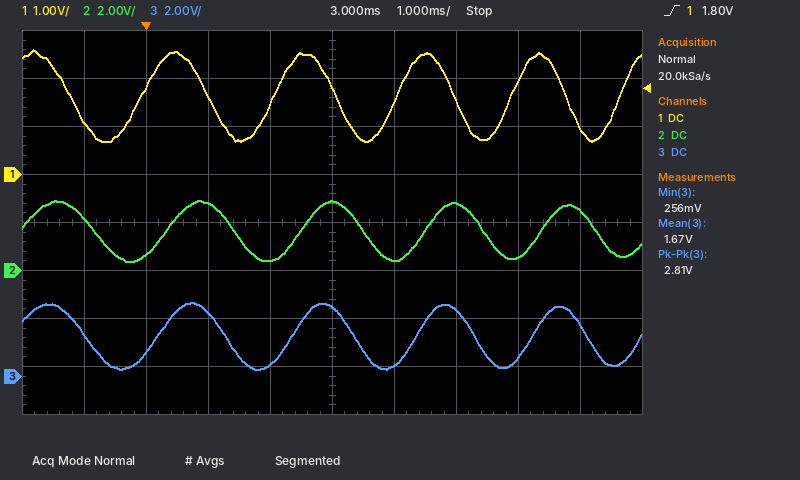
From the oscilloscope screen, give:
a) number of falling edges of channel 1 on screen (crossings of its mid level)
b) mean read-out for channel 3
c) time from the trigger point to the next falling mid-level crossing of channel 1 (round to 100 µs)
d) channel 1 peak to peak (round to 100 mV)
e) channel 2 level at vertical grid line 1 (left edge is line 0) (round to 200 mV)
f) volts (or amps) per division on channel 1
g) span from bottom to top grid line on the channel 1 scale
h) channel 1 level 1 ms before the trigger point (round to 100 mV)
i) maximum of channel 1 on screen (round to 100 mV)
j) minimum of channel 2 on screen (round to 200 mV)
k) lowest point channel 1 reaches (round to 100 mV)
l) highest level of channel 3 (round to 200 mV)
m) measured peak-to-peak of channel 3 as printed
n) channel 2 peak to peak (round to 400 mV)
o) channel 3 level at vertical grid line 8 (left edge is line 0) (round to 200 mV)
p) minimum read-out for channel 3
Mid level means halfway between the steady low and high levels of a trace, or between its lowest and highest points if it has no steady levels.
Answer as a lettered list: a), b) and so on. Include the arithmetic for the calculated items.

a) 5
b) 1.67 V
c) 1.0 ms
d) 2.6 V − (700 mV) = 1.9 V
e) 2.2 V
f) 1 V
g) 8 V
h) 1.1 V
i) 2.6 V
j) 400 mV
k) 700 mV
l) 3.0 V
m) 2.81 V
n) 2.4 V
o) 800 mV
p) 256 mV
